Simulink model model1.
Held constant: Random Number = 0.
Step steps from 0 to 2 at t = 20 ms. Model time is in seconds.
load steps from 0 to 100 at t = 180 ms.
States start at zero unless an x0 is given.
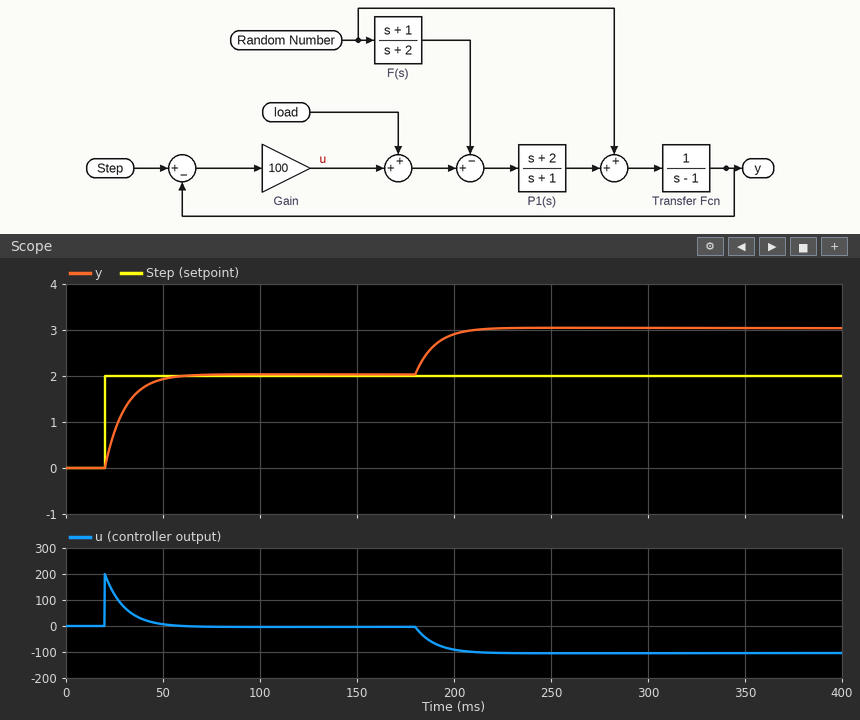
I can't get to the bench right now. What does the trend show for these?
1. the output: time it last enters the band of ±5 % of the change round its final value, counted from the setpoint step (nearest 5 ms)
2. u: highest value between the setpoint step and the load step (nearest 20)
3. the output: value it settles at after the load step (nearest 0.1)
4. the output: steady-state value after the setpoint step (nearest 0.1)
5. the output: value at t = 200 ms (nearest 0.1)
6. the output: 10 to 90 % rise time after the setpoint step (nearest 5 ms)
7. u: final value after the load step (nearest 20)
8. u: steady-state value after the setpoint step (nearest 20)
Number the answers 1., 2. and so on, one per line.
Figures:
1. 30 ms
2. 200
3. 3.0
4. 2.0
5. 2.9
6. 20 ms
7. -100
8. 0
